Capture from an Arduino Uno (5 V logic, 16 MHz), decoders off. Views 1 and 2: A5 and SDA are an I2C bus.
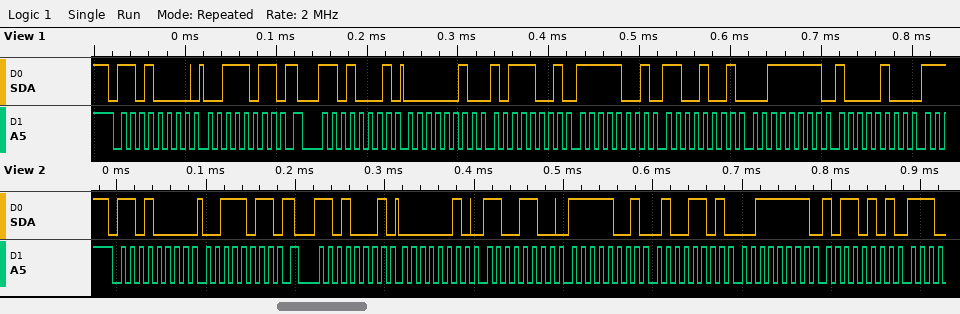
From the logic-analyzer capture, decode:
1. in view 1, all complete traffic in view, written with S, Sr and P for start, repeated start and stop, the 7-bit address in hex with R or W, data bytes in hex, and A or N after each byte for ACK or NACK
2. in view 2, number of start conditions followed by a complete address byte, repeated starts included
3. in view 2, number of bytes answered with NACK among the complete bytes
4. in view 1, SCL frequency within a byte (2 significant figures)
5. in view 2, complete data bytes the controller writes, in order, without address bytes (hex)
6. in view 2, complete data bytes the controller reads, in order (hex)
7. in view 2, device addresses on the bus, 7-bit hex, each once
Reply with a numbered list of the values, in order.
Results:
1. S 68W A 3B A Sr 68R A 02 A B9 A F9 A C9 A 3F A 84 A
2. 2
3. 0
4. 100 kHz
5. 3B
6. 02 CC F9 4D 3F B5
7. 0x68
